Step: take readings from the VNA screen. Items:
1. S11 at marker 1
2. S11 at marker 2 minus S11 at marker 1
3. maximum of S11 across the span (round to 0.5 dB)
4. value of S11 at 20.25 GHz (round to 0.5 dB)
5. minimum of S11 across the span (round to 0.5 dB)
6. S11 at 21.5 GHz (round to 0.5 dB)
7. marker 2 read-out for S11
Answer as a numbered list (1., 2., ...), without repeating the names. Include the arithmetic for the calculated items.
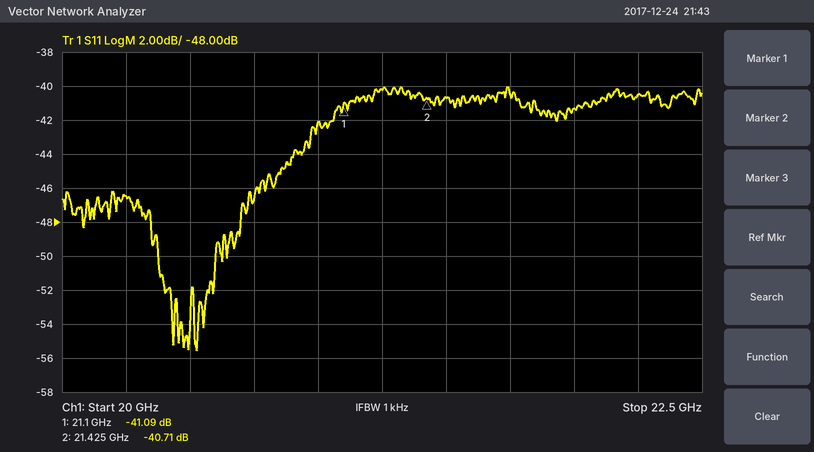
1. -41.09 dB
2. -40.71 − (-41.09) = 0.38 dB
3. -40.0 dB
4. -46.5 dB
5. -55.5 dB
6. -40.5 dB
7. -40.71 dB
